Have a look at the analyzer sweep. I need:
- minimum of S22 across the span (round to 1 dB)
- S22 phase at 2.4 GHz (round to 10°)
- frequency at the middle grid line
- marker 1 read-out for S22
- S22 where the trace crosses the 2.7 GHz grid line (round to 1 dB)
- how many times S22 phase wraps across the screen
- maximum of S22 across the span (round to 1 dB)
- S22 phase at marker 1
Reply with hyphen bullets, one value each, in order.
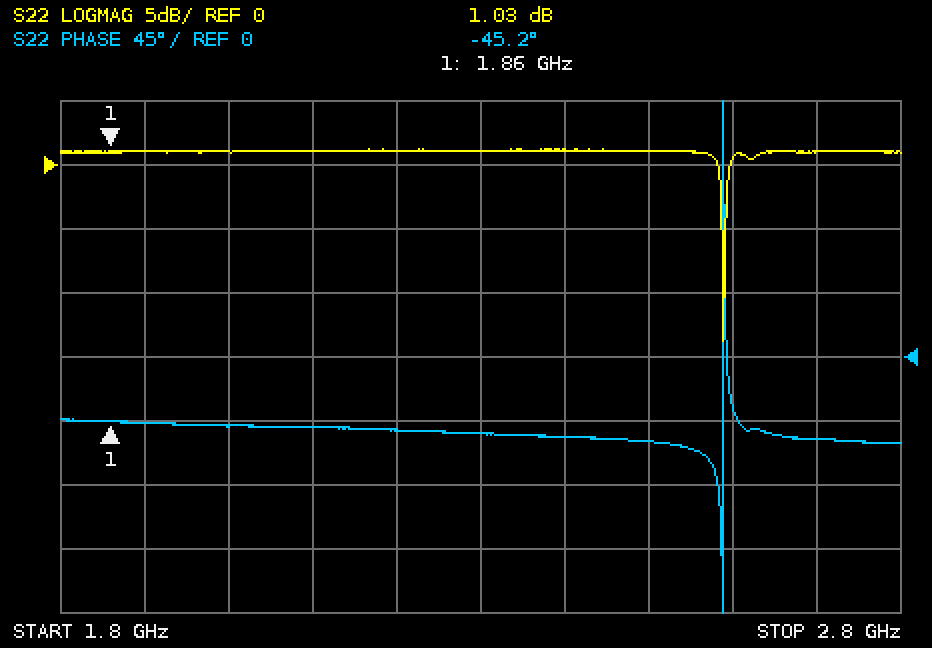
- -14 dB
- -60°
- 2.3 GHz
- 1.03 dB
- 1 dB
- 1
- 1 dB
- -45.2°
